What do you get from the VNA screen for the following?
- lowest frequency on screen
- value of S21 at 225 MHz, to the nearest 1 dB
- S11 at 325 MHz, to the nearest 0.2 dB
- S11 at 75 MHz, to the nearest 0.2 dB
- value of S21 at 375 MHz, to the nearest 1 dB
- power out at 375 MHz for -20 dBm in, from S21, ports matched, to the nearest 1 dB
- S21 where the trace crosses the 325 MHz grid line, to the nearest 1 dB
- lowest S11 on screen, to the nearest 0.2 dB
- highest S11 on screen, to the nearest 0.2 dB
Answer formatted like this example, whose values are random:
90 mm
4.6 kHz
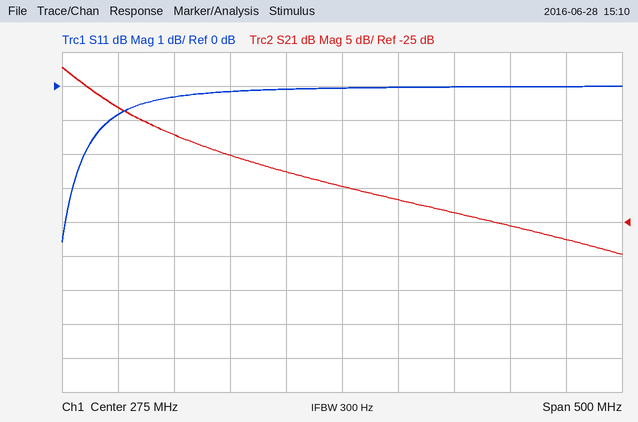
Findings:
25 MHz
-18 dB
0.0 dB
-0.8 dB
-24 dB
-44 dBm
-22 dB
-4.6 dB
0.0 dB
